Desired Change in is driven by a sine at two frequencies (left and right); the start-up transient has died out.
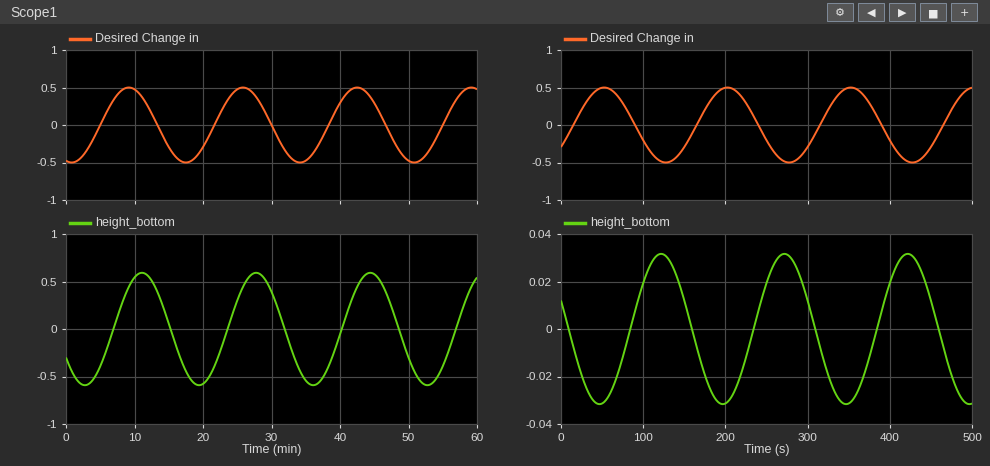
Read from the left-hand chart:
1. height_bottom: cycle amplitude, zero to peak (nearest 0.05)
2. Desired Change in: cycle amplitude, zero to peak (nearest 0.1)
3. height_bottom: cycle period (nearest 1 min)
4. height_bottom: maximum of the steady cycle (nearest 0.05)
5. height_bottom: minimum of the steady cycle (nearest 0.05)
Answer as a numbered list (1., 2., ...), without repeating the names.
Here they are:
1. 0.60
2. 0.5
3. 17 min
4. 0.60
5. -0.60
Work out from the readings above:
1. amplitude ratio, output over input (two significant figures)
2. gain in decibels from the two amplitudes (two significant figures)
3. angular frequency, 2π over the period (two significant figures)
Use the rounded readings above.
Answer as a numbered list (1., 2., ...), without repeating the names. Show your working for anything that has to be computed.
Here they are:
1. 0.6 / 0.5 = 1.2
2. 20 log10(0.6 / 0.5) = 1.6 dB
3. 2π / 17 = 0.37 rad/min
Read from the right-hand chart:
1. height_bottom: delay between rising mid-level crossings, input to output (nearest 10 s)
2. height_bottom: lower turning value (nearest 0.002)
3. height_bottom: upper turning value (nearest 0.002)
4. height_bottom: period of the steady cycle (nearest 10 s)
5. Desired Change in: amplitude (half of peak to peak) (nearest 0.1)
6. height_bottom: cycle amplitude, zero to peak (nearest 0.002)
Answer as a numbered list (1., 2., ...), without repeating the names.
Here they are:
1. 70 s
2. -0.032
3. 0.032
4. 150 s
5. 0.5
6. 0.032
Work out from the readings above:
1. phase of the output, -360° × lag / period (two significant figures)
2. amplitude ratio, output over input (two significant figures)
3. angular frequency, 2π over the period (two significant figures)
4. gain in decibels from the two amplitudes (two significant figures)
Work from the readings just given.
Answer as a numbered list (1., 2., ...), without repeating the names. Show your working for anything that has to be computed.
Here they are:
1. -360 × 70 / 150 = -170°
2. 0.032 / 0.5 = 0.064
3. 2π / 150 = 0.042 rad/s
4. 20 log10(0.032 / 0.5) = -24 dB
